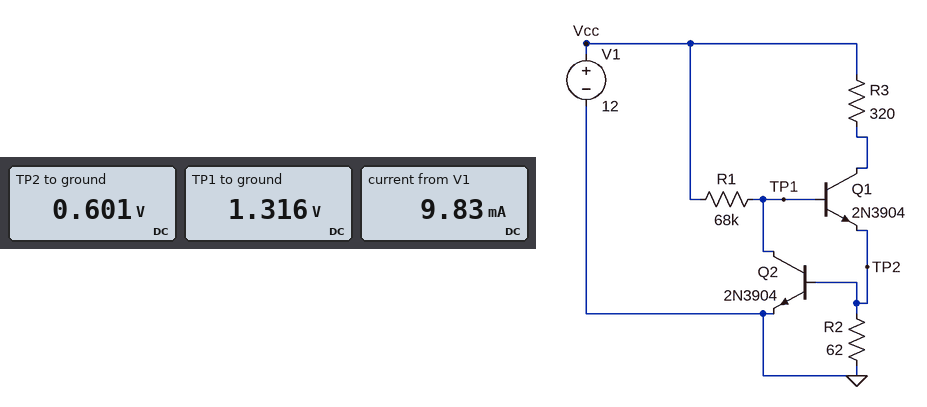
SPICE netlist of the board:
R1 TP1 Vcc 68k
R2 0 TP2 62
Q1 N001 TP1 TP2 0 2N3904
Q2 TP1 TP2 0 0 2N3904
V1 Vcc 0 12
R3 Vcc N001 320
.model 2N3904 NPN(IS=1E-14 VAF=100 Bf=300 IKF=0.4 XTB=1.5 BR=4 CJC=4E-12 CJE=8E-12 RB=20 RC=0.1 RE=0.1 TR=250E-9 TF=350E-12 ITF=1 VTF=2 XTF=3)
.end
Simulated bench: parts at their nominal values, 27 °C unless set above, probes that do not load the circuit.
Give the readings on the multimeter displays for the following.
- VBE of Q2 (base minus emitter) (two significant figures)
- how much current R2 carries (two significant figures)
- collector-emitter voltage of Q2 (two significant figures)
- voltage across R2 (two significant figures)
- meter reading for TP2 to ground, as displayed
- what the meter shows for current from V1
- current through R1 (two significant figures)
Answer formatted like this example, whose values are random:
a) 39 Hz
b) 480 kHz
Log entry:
a) 600 mV
b) 9.7 mA
c) 1.3 V
d) 600 mV
e) 0.601 V
f) 9.83 mA
g) 160 µA
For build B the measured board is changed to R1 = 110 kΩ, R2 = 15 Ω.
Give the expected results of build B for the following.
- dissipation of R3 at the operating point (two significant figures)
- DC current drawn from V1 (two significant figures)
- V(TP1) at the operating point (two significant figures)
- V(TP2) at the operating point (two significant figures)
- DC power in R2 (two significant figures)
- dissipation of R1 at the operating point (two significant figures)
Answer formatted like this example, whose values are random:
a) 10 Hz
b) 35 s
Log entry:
a) 250 mW
b) 28 mA
c) 1.2 V
d) 420 mV
e) 12 mW
f) 1.1 mW
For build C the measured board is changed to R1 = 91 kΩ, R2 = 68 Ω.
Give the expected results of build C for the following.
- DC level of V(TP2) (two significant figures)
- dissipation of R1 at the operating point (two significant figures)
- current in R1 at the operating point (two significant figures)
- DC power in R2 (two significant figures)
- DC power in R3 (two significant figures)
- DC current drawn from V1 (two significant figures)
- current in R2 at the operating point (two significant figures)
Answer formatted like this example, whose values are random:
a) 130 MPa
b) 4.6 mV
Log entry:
a) 590 mV
b) 1.3 mW
c) 120 µA
d) 5.2 mW
e) 24 mW
f) 8.8 mA
g) 8.7 mA
